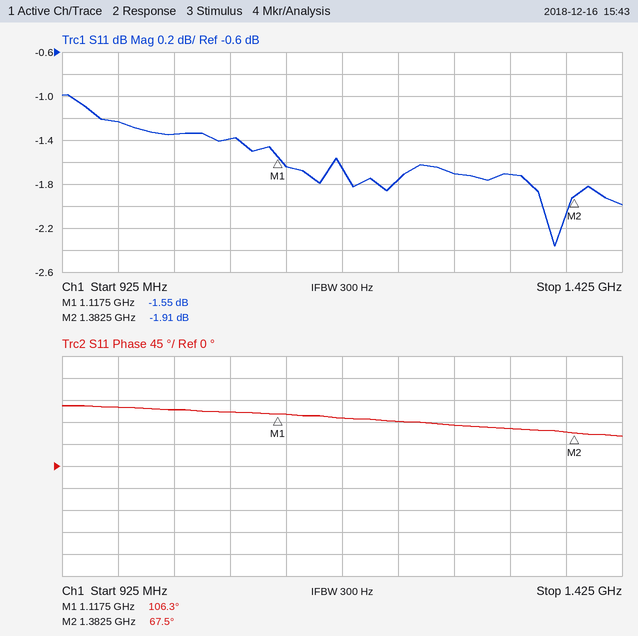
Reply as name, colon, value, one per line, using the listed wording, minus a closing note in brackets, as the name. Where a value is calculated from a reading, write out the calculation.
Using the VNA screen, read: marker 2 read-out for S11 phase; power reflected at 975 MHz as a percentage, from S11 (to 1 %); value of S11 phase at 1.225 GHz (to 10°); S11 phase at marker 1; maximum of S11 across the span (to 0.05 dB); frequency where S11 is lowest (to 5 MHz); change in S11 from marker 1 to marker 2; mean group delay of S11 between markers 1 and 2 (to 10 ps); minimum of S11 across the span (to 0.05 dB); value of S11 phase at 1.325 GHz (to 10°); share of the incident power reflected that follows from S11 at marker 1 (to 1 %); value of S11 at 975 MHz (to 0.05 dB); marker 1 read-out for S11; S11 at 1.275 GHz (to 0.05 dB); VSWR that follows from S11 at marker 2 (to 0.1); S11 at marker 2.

marker 2 read-out for S11 phase: 67.5°
power reflected at 975 MHz as a percentage, from S11: 10^(-1.25/10) ≈ 75 %
value of S11 phase at 1.225 GHz: 90°
S11 phase at marker 1: 106.3°
maximum of S11 across the span: -1.00 dB
frequency where S11 is lowest: 1.365 GHz
change in S11 from marker 1 to marker 2: -1.91 − (-1.55) = -0.36 dB
mean group delay of S11 between markers 1 and 2: −(67.5° − (106.3°))/(360° × 265 MHz) ≈ 407 ps, so 410 ps to the nearest 10 ps
minimum of S11 across the span: -2.35 dB
value of S11 phase at 1.325 GHz: 80°
share of the incident power reflected that follows from S11 at marker 1: 10^(-1.55/10) ≈ 70 %
value of S11 at 975 MHz: -1.25 dB
marker 1 read-out for S11: -1.55 dB
S11 at 1.275 GHz: -1.70 dB
VSWR that follows from S11 at marker 2: (1 + 0.8026)/(1 − 0.8026) ≈ 9.1
S11 at marker 2: -1.91 dB
